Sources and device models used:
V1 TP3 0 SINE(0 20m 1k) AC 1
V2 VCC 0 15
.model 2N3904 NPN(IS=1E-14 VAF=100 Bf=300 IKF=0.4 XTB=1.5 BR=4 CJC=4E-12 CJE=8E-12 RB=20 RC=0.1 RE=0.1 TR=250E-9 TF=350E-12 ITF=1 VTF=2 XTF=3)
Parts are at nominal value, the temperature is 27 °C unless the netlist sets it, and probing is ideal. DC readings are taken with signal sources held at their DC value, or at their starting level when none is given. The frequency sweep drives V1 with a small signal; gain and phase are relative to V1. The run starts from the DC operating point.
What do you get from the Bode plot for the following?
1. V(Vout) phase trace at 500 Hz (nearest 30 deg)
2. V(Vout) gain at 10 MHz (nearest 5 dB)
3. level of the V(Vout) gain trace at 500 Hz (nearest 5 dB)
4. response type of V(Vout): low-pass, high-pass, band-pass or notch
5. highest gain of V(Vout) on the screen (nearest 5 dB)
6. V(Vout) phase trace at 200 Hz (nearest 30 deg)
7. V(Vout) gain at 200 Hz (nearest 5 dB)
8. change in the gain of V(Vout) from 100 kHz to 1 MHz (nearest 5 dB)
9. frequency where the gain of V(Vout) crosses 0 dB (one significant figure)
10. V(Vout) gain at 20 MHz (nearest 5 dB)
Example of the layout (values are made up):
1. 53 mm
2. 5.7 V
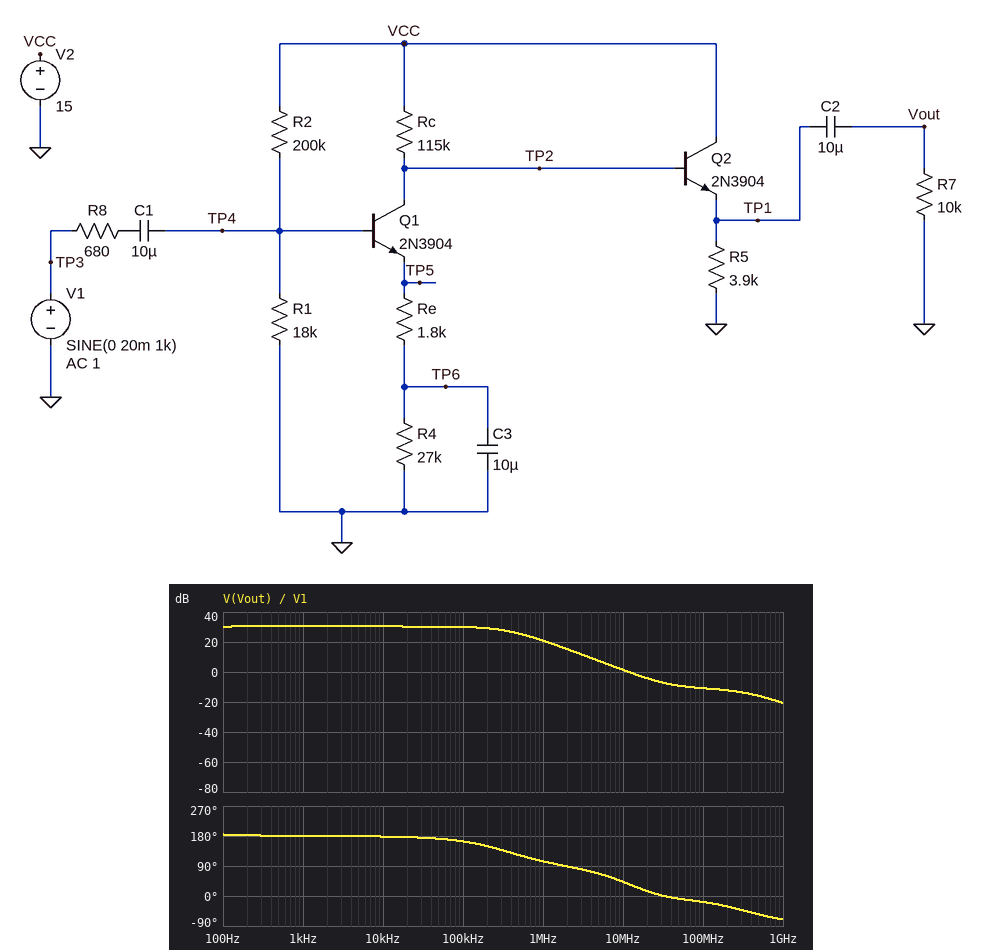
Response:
1. 180 deg
2. 0 dB
3. 30 dB
4. low-pass
5. 30 dB
6. 180 deg
7. 30 dB
8. -10 dB
9. 10 MHz
10. -5 dB
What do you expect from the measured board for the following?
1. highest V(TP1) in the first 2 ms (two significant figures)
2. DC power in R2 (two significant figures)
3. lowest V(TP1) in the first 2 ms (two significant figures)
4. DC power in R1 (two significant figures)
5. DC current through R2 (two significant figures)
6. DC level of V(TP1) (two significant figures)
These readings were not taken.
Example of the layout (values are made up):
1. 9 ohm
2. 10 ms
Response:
1. 11 V
2. 950 µW
3. 9.9 V
4. 85 µW
5. 69 µA
6. 11 V
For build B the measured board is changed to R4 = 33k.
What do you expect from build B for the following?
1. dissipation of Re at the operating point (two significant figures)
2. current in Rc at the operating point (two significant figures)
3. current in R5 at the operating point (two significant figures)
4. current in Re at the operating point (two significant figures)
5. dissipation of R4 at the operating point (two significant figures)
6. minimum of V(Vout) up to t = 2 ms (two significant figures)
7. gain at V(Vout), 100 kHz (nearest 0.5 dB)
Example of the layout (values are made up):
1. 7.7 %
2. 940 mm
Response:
1. 700 nW
2. 29 µA
3. 2.8 mA
4. 20 µA
5. 13 µW
6. -640 mV
7. 29.5 dB
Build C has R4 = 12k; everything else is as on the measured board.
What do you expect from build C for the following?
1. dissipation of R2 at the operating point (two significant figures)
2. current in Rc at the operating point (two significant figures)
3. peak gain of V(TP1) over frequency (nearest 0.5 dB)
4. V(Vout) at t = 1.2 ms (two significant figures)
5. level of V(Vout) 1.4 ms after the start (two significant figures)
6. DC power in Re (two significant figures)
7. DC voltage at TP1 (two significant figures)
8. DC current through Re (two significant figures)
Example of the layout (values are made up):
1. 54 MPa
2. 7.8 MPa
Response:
1. 950 µW
2. 54 µA
3. 32.0 dB
4. -780 mV
5. -470 mV
6. 4.1 µW
7. 8.1 V
8. 48 µA
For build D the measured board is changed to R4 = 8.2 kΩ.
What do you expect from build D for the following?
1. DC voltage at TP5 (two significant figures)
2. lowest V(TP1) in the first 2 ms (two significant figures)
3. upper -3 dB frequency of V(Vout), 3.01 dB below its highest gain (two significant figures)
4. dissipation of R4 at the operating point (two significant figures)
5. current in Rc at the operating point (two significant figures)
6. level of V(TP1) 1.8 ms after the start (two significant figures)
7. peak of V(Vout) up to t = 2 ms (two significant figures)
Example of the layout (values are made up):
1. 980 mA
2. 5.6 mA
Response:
1. 650 mV
2. 5.4 V
3. 350 kHz
4. 35 µW
5. 70 µA
6. 7.1 V
7. 870 mV
